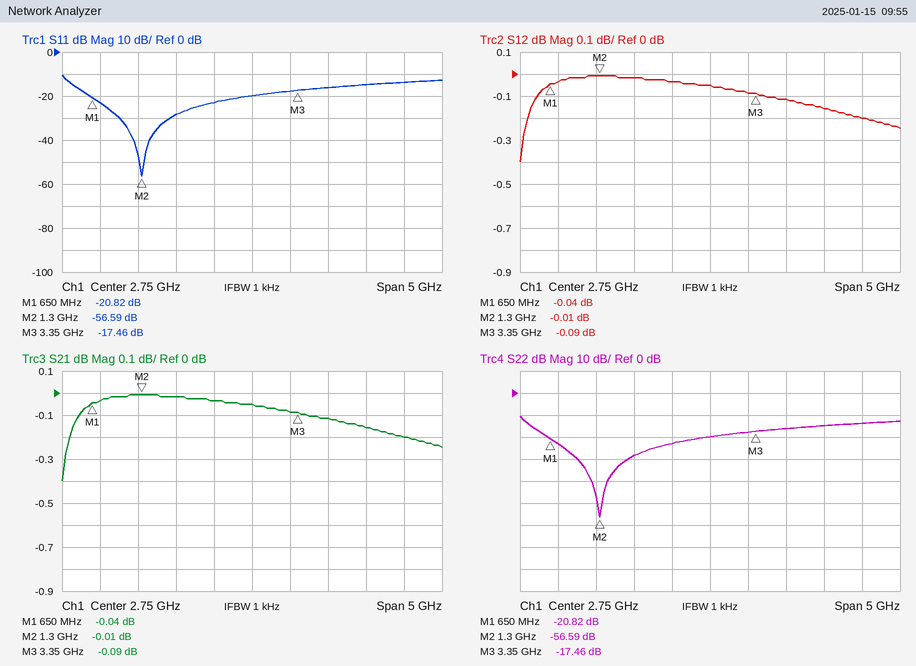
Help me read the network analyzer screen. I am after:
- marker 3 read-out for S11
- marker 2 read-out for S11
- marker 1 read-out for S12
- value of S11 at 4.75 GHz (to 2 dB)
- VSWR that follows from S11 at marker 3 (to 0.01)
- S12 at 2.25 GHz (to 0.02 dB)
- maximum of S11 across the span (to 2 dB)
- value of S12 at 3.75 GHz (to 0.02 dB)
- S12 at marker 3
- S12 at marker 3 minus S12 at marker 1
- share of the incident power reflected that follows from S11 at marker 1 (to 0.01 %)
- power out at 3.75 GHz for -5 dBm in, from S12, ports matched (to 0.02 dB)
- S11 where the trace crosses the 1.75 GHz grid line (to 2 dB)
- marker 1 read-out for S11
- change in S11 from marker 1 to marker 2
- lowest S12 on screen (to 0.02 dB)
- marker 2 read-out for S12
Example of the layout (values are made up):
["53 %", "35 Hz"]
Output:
["-17.46 dB", "-56.59 dB", "-0.04 dB", "-14 dB", "1.31", "-0.04 dB", "-10 dB", "-0.12 dB", "-0.09 dB", "-0.05 dB", "0.83 %", "-5.12 dBm", "-28 dB", "-20.82 dB", "-35.77 dB", "-0.40 dB", "-0.01 dB"]
